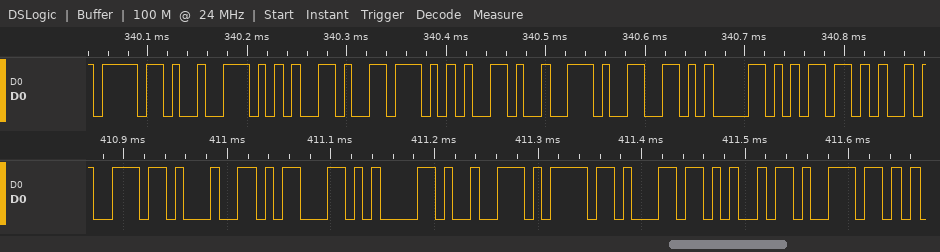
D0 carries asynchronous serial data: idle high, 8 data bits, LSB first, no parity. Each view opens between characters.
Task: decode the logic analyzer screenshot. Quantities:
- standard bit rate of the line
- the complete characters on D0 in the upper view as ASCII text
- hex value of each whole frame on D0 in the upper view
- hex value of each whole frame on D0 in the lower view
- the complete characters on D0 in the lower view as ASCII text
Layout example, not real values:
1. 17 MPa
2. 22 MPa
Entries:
1. 115200 baud
2. "oreverfam"
3. 6F, 72, 65, 76, 65, 72, 66, 61, 6D
4. 6E, 64, 63, 61, 72, 6F, 6C, 69, 6E
5. "ndcarolin"
